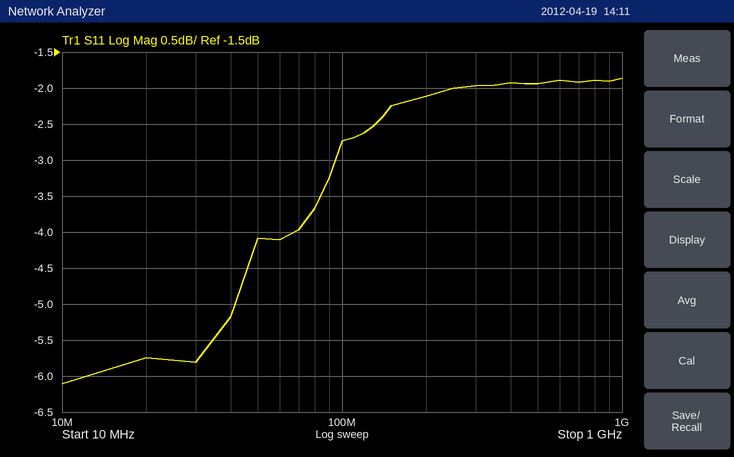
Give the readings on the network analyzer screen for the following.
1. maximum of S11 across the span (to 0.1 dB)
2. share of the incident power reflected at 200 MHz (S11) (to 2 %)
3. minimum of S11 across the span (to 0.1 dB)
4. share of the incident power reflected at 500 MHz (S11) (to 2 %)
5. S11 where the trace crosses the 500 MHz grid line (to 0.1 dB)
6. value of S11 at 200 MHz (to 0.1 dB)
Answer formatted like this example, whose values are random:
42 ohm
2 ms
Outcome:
-1.9 dB
62 %
-6.1 dB
64 %
-1.9 dB
-2.1 dB
